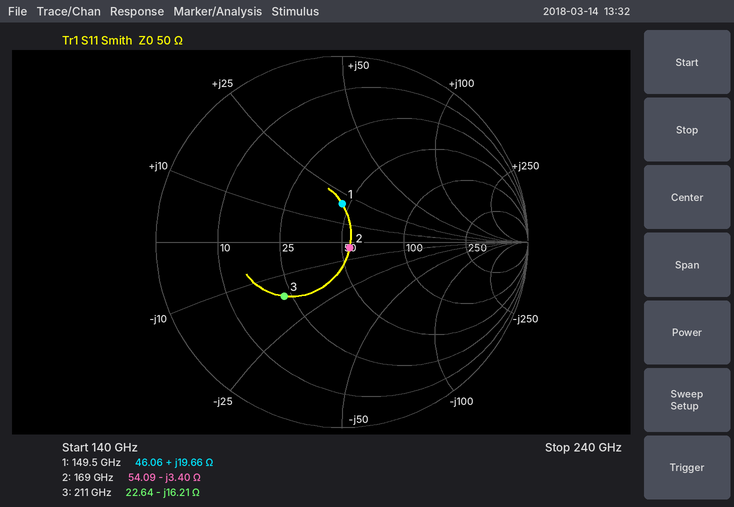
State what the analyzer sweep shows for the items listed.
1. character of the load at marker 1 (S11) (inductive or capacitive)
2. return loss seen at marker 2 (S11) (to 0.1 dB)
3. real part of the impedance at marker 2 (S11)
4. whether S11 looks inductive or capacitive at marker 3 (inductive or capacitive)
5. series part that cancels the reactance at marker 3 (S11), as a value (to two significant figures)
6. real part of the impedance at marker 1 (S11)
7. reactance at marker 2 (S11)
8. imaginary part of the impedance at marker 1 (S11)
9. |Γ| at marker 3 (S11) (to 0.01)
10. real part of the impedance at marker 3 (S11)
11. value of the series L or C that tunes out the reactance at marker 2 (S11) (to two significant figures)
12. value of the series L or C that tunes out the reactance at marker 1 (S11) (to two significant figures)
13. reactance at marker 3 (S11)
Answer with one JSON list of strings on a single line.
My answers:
["inductive", "25.8 dB", "54.09 Ω", "capacitive", "12 pH", "46.06 Ω", "-3.40 Ω", "+19.66 Ω", "0.43", "22.64 Ω", "3.2 pH", "54 fF", "-16.21 Ω"]
